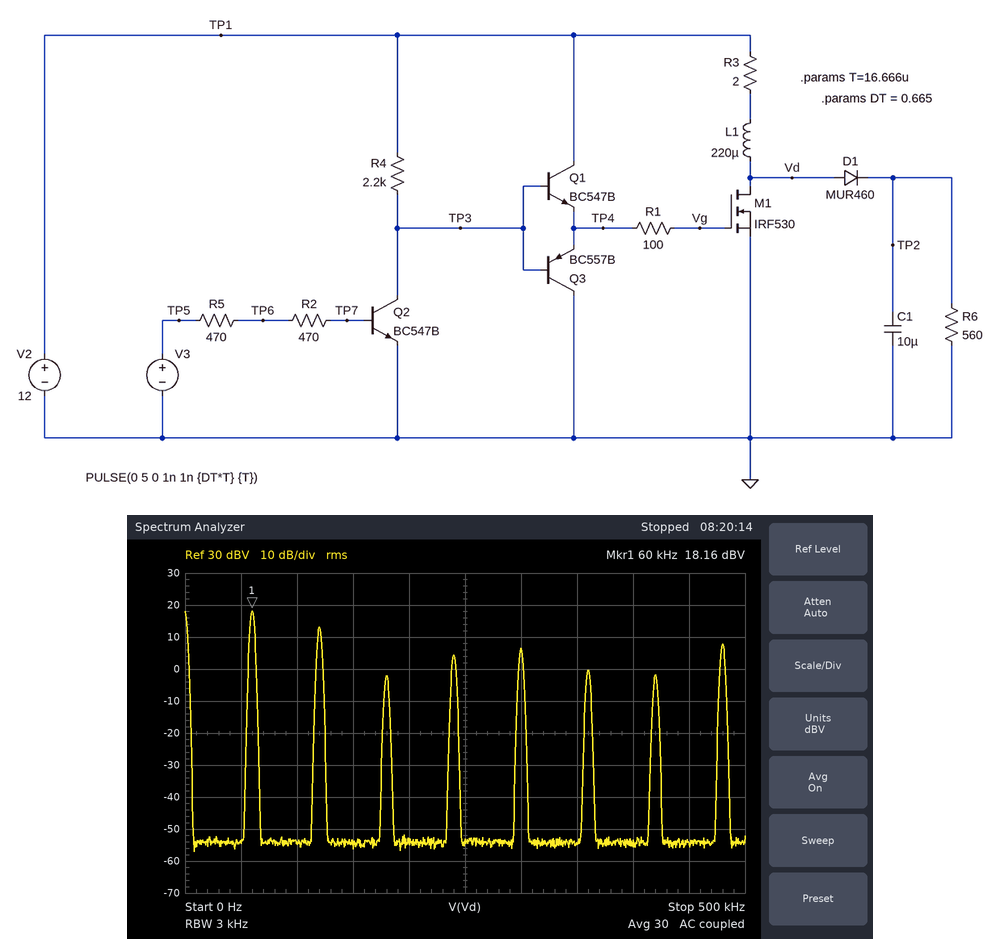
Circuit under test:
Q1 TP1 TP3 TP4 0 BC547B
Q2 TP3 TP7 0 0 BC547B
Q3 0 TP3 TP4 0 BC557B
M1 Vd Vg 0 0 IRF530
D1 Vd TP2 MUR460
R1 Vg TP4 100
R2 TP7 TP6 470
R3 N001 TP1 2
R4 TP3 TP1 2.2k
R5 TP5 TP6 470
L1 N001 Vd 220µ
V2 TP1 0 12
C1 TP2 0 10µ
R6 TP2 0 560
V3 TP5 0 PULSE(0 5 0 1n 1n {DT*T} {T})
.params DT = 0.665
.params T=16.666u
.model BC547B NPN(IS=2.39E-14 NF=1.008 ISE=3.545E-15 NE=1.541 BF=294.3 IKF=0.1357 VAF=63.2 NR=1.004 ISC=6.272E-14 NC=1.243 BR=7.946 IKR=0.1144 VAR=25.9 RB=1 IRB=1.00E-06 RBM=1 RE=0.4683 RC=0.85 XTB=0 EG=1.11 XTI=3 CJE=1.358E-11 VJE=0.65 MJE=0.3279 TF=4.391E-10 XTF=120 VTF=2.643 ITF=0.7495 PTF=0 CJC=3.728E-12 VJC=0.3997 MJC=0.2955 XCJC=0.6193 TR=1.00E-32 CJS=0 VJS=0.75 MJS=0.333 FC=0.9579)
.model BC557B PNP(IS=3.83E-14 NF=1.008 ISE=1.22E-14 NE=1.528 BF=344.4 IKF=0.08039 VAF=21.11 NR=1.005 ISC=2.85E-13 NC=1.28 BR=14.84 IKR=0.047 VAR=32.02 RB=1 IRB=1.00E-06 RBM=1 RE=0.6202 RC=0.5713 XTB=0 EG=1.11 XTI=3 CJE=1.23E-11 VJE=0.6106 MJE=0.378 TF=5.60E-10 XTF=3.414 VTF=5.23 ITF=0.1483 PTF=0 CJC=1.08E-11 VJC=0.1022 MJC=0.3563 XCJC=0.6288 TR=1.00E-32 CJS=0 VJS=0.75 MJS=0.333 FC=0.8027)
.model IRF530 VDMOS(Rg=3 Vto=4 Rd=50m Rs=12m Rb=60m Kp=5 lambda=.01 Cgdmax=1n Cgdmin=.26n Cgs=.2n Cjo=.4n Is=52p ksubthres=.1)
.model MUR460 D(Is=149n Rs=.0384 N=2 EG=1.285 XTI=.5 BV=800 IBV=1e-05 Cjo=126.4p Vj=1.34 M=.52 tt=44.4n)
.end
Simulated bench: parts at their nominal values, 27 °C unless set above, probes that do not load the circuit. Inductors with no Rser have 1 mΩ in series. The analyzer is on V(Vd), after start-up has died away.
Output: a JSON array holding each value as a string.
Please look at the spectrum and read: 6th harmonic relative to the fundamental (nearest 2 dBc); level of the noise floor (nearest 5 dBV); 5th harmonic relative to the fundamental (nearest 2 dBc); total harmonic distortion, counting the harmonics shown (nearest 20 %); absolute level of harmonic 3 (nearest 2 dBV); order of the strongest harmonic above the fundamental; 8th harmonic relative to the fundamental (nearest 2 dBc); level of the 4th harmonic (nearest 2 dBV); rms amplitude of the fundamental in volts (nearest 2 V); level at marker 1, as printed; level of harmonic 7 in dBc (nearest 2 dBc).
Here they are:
["-18 dBc", "-55 dBV", "-12 dBc", "80 %", "-2 dBV", "2", "-10 dBc", "4 dBV", "8 V", "18.16 dBV", "-20 dBc"]
